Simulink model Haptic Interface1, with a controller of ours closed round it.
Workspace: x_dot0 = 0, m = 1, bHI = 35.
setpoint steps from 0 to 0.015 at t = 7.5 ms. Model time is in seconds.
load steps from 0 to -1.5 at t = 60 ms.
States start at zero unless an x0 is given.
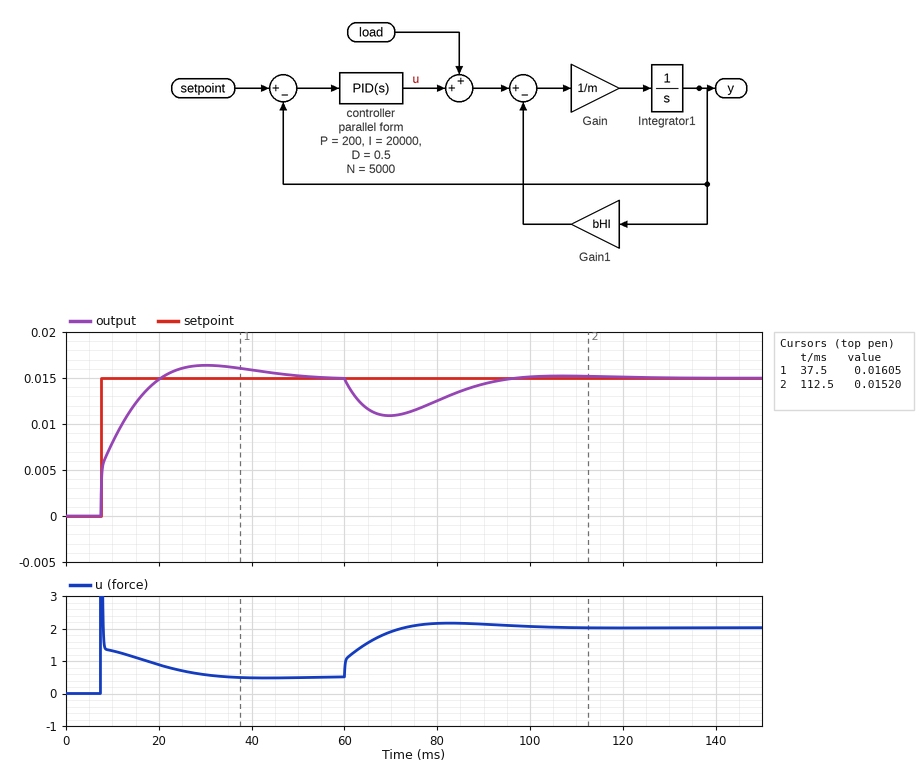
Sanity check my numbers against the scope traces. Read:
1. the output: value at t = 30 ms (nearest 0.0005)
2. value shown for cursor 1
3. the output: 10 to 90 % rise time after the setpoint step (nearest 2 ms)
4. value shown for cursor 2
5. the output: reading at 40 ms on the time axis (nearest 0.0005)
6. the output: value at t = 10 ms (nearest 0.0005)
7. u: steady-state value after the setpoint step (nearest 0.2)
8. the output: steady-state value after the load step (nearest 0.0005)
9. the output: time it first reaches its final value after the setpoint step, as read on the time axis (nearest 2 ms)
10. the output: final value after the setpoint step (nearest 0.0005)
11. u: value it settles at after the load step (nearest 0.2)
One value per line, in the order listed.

0.0165
0.01605
10 ms
0.01520
0.0160
0.0080
0.6
0.0150
20 ms
0.0150
2.0
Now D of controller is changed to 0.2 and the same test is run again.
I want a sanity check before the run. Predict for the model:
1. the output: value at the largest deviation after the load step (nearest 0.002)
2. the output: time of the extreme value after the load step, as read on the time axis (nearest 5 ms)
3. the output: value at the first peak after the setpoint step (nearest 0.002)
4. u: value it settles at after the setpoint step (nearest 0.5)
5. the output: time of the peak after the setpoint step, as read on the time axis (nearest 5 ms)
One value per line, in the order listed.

0.010
70 ms
0.016
0.5
25 ms
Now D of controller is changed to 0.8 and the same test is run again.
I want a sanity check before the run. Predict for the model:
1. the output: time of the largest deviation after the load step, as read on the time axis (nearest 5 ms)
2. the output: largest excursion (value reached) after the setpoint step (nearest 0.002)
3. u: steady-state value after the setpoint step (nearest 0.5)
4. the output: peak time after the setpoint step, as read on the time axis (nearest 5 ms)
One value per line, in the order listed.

70 ms
0.016
0.5
35 ms
